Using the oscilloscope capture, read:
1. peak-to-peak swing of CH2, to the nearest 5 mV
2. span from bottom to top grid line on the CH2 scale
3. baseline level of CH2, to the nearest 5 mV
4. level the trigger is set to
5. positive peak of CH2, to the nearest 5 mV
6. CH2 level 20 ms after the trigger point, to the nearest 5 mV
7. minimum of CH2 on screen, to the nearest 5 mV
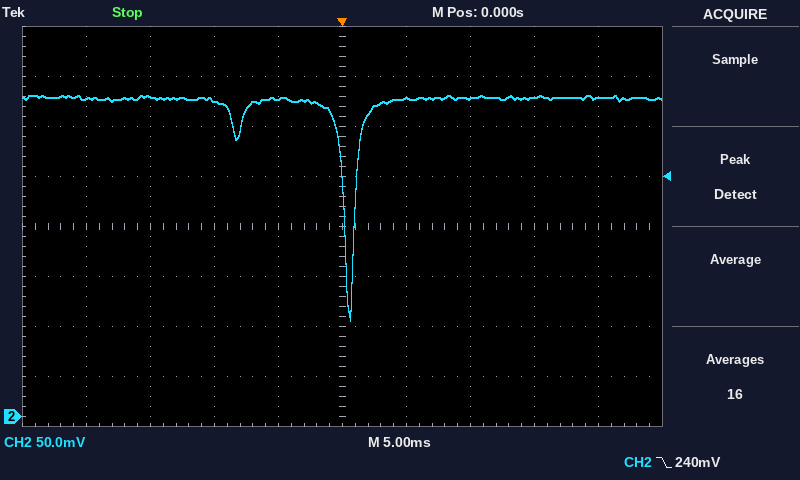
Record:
225 mV
400 mV
320 mV
240 mV
320 mV
320 mV
95 mV
